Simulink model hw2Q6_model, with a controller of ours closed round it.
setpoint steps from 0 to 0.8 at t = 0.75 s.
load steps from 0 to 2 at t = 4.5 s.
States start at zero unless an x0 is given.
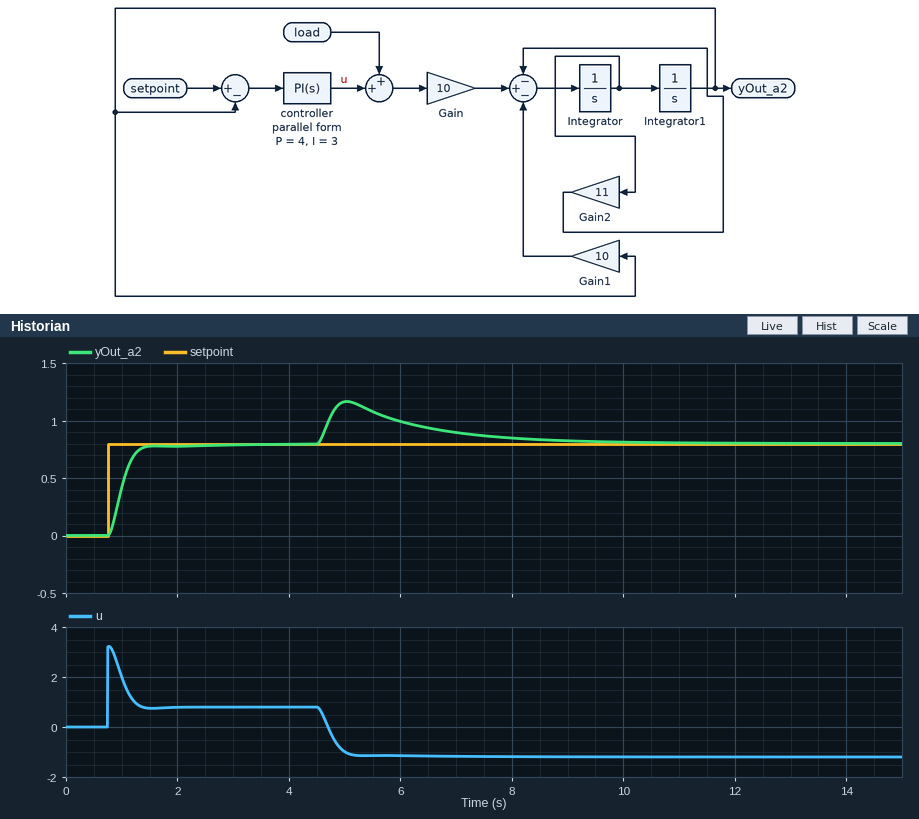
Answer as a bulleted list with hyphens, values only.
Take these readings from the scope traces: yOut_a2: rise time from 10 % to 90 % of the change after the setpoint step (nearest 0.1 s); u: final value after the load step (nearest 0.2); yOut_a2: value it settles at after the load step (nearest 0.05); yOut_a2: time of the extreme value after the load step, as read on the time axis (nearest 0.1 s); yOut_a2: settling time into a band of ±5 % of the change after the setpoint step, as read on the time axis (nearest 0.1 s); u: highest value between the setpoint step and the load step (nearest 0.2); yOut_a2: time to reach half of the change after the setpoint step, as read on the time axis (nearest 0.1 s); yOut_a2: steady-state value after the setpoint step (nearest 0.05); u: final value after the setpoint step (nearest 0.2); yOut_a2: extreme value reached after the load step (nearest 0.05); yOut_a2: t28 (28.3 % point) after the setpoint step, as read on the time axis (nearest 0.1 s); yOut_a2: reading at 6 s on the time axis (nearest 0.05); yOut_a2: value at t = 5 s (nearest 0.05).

- 0.4 s
- -1.2
- 0.80
- 5.0 s
- 1.4 s
- 3.2
- 1.0 s
- 0.80
- 0.8
- 1.15
- 0.9 s
- 1.00
- 1.15
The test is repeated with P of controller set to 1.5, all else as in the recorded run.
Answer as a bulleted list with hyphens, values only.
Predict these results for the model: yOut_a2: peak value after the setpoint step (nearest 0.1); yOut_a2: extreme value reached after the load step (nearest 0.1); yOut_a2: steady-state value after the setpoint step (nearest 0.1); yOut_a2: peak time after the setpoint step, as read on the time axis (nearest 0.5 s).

- 0.9
- 1.4
- 0.8
- 2.5 s
